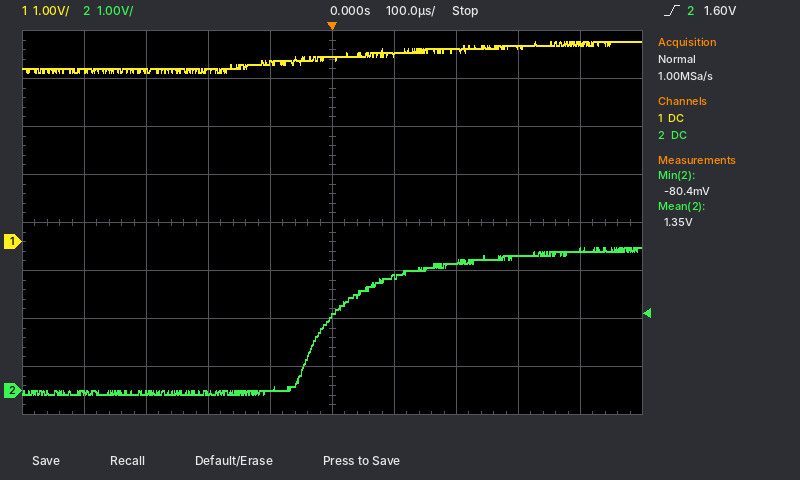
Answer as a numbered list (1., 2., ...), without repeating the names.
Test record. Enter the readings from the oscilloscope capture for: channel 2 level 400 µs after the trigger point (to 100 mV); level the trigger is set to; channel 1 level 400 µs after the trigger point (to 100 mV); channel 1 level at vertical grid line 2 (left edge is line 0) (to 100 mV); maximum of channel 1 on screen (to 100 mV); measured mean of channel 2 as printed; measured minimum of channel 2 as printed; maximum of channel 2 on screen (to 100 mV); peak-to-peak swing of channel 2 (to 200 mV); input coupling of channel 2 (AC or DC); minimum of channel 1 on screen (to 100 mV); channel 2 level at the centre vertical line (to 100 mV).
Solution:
1. 2.9 V
2. 1.60 V
3. 4.1 V
4. 3.6 V
5. 4.2 V
6. 1.35 V
7. -80.4 mV
8. 3.0 V
9. 3.0 V
10. DC
11. 3.5 V
12. 1.5 V
